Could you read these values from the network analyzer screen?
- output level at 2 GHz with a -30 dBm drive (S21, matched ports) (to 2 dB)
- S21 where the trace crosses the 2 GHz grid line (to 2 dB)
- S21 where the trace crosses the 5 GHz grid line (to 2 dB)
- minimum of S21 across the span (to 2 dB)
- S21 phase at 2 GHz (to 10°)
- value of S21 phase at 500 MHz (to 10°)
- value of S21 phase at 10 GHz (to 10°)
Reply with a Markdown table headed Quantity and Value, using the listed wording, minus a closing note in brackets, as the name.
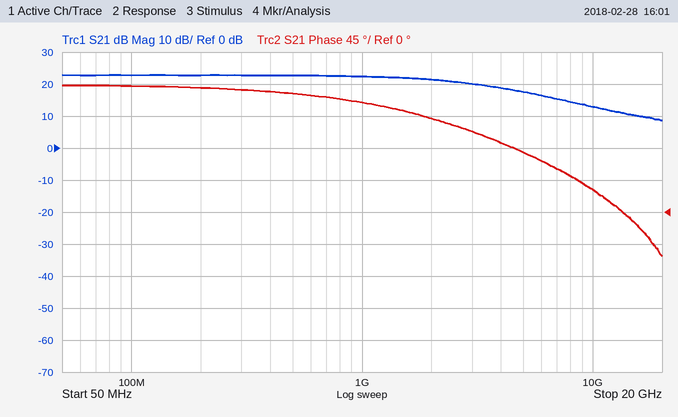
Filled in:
| Quantity | Value |
|---|---|
| output level at 2 GHz with a -30 dBm drive (S21, matched ports) | -8 dBm |
| S21 where the trace crosses the 2 GHz grid line | 22 dB |
| S21 where the trace crosses the 5 GHz grid line | 18 dB |
| minimum of S21 across the span | 8 dB |
| S21 phase at 2 GHz | 130° |
| value of S21 phase at 500 MHz | 170° |
| value of S21 phase at 10 GHz | 30° |
